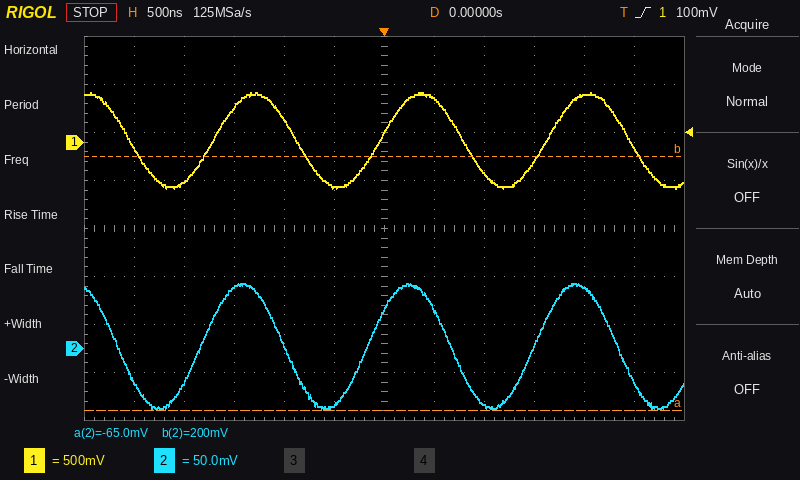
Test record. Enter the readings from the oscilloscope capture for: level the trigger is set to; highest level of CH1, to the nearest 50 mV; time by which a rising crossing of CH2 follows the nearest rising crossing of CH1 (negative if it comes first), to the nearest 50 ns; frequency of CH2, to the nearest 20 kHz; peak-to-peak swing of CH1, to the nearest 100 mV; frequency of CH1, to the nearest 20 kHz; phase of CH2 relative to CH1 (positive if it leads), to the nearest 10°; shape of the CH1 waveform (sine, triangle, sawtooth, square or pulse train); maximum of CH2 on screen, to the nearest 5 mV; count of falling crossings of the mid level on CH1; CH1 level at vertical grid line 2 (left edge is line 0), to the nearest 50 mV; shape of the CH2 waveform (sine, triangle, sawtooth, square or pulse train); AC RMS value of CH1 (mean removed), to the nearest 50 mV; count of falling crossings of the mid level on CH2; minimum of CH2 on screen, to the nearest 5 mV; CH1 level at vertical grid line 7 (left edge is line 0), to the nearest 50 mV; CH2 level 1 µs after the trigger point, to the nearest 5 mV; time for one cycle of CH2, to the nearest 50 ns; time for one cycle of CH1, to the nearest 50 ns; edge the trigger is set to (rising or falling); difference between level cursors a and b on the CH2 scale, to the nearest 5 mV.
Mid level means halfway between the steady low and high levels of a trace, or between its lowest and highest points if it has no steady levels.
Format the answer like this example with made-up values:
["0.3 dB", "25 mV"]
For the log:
["100 mV", "500 mV", "-150 ns", "600 kHz", "1.00 V", "600 kHz", "+30°", "sine", "70 mV", "4", "-400 mV", "sine", "350 mV", "4", "-65 mV", "450 mV", "-60 mV", "1.65 µs", "1.65 µs", "rising", "265 mV"]
